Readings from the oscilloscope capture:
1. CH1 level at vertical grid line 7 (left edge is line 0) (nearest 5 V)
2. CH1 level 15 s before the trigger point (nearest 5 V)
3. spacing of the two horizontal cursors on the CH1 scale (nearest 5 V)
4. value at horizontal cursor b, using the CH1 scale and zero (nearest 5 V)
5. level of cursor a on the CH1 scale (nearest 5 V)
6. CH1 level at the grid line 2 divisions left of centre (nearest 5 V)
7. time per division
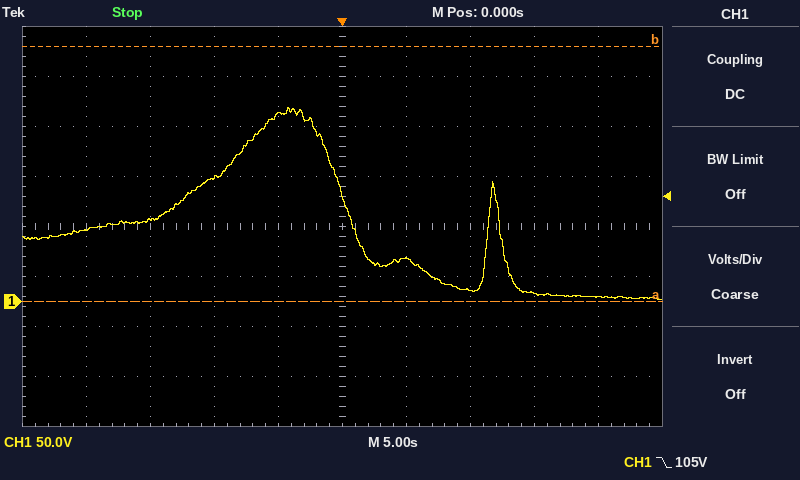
10 V
80 V
255 V
255 V
0 V
125 V
5 s
